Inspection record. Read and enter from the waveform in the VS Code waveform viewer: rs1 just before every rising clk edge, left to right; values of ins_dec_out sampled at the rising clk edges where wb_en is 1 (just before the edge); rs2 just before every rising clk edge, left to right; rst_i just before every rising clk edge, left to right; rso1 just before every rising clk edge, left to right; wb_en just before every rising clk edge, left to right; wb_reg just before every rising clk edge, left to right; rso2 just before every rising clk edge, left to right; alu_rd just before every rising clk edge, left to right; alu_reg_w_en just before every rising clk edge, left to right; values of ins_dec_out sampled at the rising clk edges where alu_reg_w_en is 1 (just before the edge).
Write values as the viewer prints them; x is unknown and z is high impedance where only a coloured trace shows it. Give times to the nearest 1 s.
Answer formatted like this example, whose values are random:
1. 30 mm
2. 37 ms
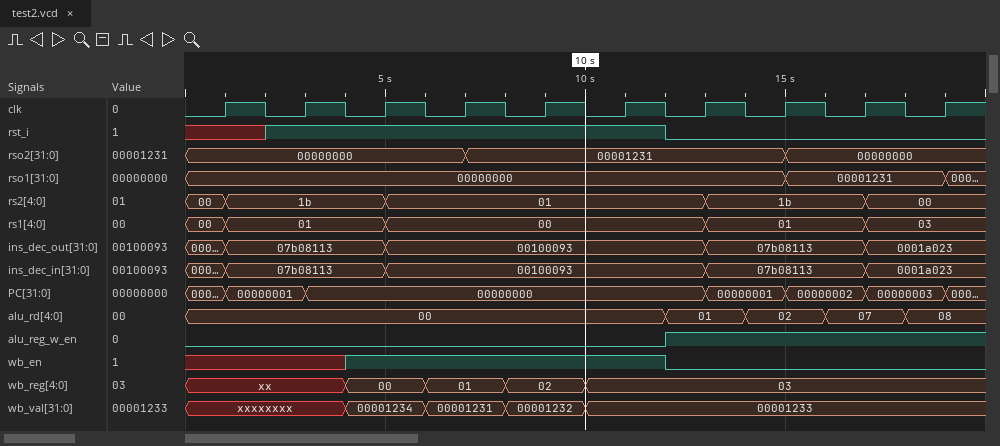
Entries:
1. 00, 01, 01, 00, 00, 00, 00, 01, 01, 03
2. 07b08113, 00100093, 00100093, 00100093
3. 00, 1b, 1b, 01, 01, 01, 01, 1b, 1b, 00
4. x 1 1 1 1 1 0 0 0 0
5. 00000000, 00000000, 00000000, 00000000, 00000000, 00000000, 00000000, 00000000, 00001231, 00001231
6. x x 1 1 1 1 0 0 0 0
7. xx, xx, 00, 01, 02, 03, 03, 03, 03, 03
8. 00000000, 00000000, 00000000, 00000000, 00001231, 00001231, 00001231, 00001231, 00000000, 00000000
9. 00, 00, 00, 00, 00, 00, 01, 02, 07, 08
10. 0 0 0 0 0 0 1 1 1 1
11. 00100093, 07b08113, 07b08113, 0001a023
